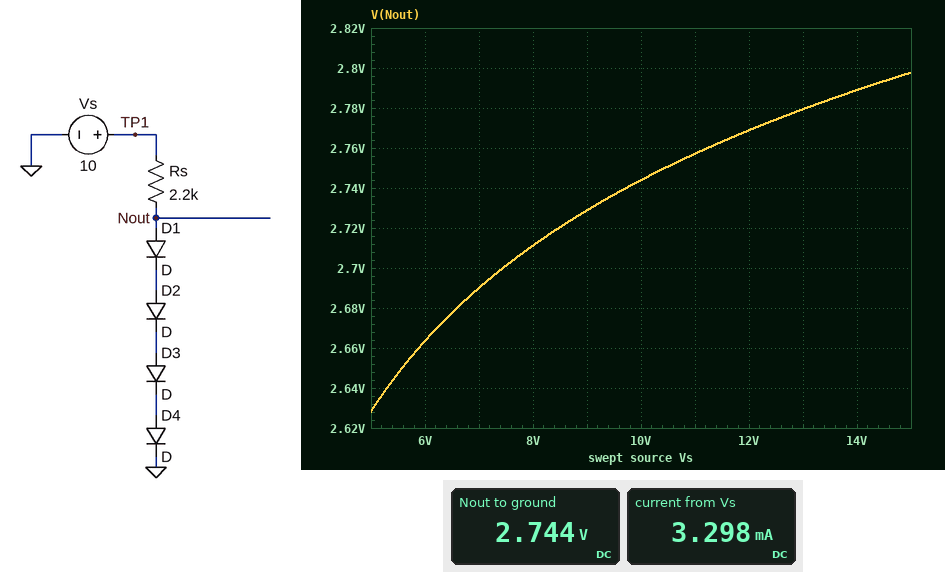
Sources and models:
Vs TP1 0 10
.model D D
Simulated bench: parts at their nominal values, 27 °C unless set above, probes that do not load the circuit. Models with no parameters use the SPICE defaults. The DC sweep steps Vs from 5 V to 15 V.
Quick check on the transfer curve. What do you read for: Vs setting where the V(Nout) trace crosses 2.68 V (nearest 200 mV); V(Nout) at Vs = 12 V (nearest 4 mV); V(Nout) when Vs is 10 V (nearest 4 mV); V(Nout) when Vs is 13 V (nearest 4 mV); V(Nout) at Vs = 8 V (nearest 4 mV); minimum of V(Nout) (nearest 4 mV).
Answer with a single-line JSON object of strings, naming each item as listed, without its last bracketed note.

{"Vs setting where the V(Nout) trace crosses 2.68 V": "6.6 V", "V(Nout) at Vs = 12 V": "2.768 V", "V(Nout) when Vs is 10 V": "2.744 V", "V(Nout) when Vs is 13 V": "2.780 V", "V(Nout) at Vs = 8 V": "2.712 V", "minimum of V(Nout)": "2.628 V"}
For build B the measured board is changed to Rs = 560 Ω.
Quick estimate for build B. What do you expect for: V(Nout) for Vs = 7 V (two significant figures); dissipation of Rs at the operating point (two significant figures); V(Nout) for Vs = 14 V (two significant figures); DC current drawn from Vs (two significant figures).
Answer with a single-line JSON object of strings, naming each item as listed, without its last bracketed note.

{"V(Nout) for Vs = 7 V": "2.8 V", "dissipation of Rs at the operating point": "90 mW", "V(Nout) for Vs = 14 V": "2.9 V", "DC current drawn from Vs": "13 mA"}
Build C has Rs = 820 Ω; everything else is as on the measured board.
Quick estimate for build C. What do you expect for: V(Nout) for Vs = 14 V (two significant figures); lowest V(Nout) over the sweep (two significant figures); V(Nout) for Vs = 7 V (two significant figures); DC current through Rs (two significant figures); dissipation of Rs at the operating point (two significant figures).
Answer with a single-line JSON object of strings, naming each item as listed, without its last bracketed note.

{"V(Nout) for Vs = 14 V": "2.9 V", "lowest V(Nout) over the sweep": "2.7 V", "V(Nout) for Vs = 7 V": "2.8 V", "DC current through Rs": "8.7 mA", "dissipation of Rs at the operating point": "62 mW"}
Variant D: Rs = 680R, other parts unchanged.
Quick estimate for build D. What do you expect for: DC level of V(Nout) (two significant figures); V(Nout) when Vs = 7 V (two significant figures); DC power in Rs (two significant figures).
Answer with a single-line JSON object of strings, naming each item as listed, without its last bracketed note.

{"DC level of V(Nout)": "2.9 V", "V(Nout) when Vs = 7 V": "2.8 V", "DC power in Rs": "75 mW"}
